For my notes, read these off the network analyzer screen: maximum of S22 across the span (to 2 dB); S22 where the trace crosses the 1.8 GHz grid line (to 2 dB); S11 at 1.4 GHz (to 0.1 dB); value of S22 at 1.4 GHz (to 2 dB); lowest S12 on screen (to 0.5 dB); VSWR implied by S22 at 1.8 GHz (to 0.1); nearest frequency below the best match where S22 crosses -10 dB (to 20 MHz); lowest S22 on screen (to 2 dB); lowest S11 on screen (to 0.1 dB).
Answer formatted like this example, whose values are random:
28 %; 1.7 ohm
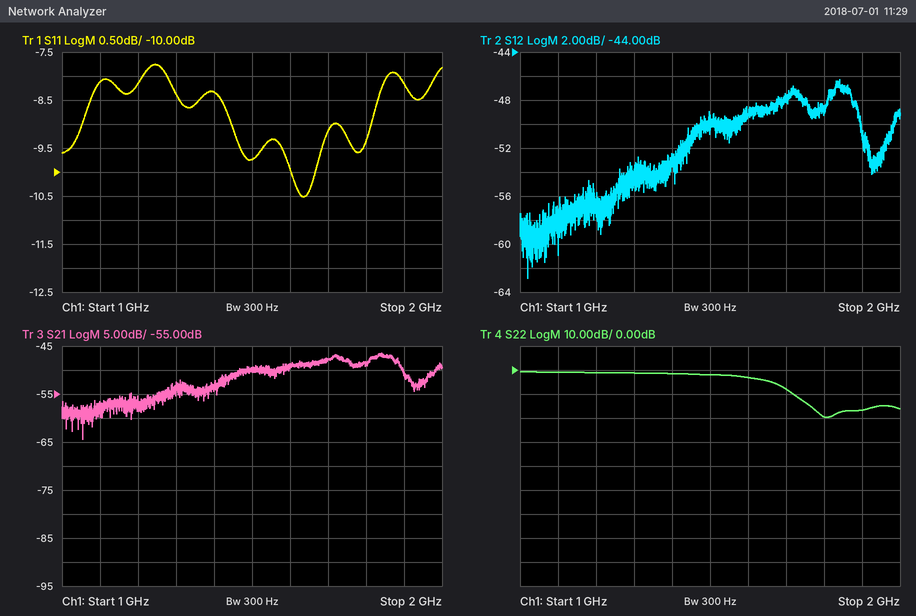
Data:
0 dB; -20 dB; -8.3 dB; -2 dB; -63.0 dB; 1.2; 1.72 GHz; -20 dB; -10.5 dB
